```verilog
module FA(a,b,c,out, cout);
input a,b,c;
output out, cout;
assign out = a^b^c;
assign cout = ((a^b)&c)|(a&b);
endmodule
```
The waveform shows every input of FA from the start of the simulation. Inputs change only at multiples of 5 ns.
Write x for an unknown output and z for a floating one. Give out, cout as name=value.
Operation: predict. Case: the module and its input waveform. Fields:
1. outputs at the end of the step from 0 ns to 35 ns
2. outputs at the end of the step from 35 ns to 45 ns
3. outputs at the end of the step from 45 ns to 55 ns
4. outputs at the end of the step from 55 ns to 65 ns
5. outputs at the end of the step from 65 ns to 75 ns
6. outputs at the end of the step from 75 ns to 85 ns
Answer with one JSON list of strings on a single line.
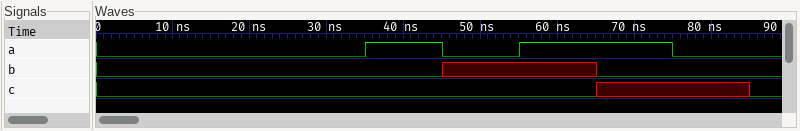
["out=0, cout=0", "out=1, cout=0", "out=x, cout=0", "out=x, cout=x", "out=x, cout=x", "out=x, cout=0"]
